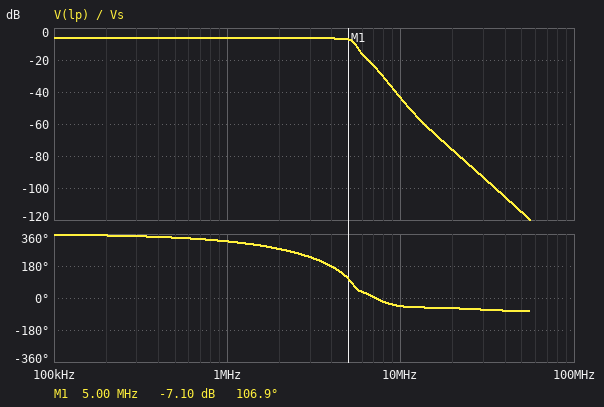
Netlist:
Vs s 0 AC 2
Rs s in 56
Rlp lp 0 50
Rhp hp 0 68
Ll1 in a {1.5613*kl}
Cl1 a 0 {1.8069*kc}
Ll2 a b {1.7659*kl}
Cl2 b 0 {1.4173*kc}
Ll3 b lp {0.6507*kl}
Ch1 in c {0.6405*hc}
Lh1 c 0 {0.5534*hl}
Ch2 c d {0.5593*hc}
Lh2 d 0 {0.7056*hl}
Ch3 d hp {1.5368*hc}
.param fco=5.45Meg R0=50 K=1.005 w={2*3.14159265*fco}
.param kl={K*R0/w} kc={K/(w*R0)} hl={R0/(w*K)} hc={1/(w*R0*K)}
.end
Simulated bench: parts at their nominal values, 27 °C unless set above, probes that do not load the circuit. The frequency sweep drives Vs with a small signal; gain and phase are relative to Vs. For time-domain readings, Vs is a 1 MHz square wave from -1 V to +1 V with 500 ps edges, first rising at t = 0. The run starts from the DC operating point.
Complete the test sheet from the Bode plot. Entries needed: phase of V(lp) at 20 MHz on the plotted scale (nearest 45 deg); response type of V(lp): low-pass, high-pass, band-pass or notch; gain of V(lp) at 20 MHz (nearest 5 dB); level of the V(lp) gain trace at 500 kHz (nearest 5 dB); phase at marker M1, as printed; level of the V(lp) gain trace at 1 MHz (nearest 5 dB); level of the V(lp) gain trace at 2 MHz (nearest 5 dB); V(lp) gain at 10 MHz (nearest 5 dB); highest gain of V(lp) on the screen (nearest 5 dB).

-45 deg
low-pass
-75 dB
-5 dB
106.9 deg
-5 dB
-5 dB
-45 dB
-5 dB
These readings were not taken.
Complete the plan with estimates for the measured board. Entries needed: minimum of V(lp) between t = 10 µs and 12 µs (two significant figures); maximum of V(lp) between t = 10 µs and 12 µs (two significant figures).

-630 mV
630 mV
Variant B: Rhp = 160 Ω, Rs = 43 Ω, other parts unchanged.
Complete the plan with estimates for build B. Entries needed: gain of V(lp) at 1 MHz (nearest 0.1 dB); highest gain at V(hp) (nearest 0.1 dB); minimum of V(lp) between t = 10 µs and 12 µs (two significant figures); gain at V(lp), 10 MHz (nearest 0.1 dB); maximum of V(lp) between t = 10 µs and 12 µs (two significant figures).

-5.4 dB
-1.3 dB
-720 mV
-42.2 dB
720 mV
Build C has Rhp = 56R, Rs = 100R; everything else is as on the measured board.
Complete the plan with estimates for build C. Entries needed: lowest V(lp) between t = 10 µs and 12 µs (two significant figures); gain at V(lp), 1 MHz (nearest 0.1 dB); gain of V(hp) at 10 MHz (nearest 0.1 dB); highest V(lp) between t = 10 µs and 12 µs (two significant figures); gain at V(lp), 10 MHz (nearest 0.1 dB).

-440 mV
-9.5 dB
-9.1 dB
440 mV
-46.7 dB
